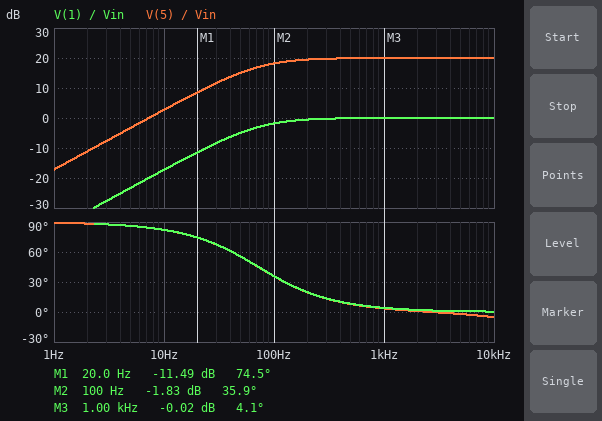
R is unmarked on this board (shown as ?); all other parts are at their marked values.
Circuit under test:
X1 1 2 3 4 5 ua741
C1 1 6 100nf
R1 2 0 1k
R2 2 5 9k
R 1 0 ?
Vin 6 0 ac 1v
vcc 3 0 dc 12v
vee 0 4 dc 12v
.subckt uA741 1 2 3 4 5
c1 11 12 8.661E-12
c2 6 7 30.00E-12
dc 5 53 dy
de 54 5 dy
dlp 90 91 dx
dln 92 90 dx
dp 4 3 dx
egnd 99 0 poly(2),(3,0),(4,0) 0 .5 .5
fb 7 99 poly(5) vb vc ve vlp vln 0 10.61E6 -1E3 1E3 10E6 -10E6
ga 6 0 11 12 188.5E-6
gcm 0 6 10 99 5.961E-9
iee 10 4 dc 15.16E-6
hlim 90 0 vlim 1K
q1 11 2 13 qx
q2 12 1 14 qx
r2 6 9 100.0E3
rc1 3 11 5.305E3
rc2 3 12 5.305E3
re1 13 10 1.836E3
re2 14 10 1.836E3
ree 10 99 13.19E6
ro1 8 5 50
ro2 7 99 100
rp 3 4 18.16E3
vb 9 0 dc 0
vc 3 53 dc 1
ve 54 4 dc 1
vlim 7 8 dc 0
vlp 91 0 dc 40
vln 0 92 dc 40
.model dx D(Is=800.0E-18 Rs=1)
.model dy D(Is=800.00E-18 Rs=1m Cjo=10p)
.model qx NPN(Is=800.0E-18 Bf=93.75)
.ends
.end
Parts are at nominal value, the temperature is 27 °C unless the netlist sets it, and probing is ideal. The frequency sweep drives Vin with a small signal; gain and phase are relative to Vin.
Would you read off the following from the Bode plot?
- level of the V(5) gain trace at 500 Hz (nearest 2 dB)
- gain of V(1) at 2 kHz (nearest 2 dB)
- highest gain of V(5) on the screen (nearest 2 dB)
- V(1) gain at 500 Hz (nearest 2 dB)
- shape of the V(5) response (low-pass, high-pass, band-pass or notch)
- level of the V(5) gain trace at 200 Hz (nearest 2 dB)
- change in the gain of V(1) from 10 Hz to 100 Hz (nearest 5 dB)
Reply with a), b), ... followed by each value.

a) 20 dB
b) 0 dB
c) 20 dB
d) 0 dB
e) high-pass
f) 20 dB
g) 15 dB
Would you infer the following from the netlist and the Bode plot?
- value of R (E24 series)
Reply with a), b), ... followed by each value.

a) 22 kΩ
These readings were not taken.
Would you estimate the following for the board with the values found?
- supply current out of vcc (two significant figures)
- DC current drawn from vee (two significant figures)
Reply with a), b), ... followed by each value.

a) 1.3 mA
b) 1.3 mA
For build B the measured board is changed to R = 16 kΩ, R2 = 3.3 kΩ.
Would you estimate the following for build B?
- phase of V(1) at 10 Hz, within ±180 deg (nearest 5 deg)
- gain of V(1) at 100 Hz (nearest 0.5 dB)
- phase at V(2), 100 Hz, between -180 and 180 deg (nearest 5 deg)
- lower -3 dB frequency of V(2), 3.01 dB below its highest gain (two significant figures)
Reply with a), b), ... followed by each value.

a) 85 deg
b) -3.0 dB
c) 45 deg
d) 99 Hz
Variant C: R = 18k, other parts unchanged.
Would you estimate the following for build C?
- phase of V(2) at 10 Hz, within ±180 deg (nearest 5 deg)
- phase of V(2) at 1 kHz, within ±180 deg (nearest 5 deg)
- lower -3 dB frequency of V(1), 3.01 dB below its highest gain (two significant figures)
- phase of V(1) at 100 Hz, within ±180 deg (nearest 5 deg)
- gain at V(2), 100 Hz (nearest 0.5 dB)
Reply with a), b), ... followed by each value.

a) 85 deg
b) 5 deg
c) 88 Hz
d) 40 deg
e) -2.5 dB
